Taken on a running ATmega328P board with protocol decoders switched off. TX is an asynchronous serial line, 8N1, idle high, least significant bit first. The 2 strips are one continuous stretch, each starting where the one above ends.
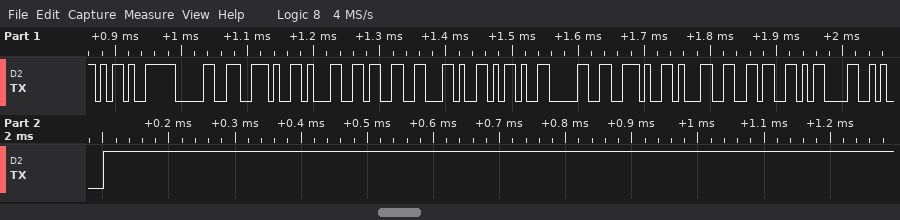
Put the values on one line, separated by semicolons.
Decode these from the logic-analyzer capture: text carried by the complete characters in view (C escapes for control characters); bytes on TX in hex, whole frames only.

"-0.13,-0.16\r\n"; 2D 30 2E 31 33 2C 2D 30 2E 31 36 0D 0A
